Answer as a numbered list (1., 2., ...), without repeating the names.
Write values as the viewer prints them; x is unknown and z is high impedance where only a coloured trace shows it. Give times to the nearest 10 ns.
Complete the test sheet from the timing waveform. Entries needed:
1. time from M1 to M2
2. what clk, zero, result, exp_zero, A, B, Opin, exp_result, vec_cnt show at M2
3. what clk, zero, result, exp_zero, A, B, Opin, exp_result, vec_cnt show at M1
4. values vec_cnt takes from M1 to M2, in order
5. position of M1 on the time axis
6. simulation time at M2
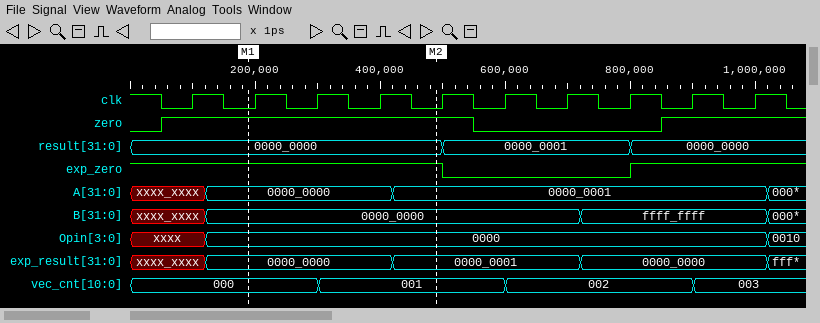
1. 300 ns
2. clk=0, zero=1, result=0000_0000, exp_zero=1, A=0000_0001, B=0000_0000, Opin=0000, exp_result=0000_0001, vec_cnt=001
3. clk=0, zero=1, result=0000_0000, exp_zero=1, A=0000_0000, B=0000_0000, Opin=0000, exp_result=0000_0000, vec_cnt=000
4. 000, 001
5. 190 ns
6. 490 ns
